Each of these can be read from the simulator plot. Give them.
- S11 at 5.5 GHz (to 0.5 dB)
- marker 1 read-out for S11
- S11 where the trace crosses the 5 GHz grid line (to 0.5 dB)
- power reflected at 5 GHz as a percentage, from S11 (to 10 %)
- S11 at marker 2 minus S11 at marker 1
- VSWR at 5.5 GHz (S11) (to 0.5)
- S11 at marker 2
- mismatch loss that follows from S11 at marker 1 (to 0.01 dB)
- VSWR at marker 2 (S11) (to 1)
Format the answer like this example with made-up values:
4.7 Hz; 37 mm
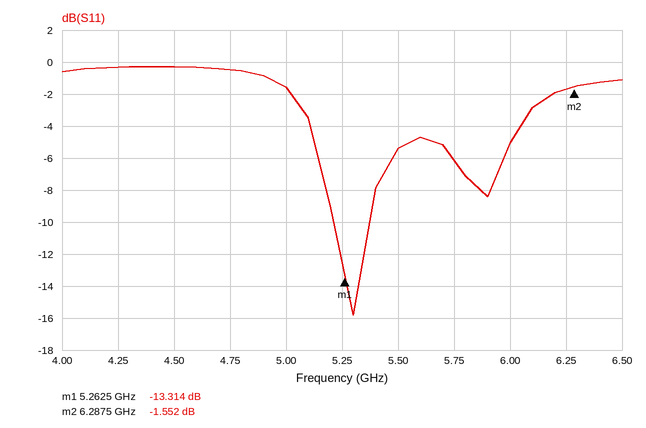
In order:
-5.5 dB; -13.314 dB; -1.5 dB; 70 %; 11.762 dB; 3.5; -1.552 dB; 0.21 dB; 11
